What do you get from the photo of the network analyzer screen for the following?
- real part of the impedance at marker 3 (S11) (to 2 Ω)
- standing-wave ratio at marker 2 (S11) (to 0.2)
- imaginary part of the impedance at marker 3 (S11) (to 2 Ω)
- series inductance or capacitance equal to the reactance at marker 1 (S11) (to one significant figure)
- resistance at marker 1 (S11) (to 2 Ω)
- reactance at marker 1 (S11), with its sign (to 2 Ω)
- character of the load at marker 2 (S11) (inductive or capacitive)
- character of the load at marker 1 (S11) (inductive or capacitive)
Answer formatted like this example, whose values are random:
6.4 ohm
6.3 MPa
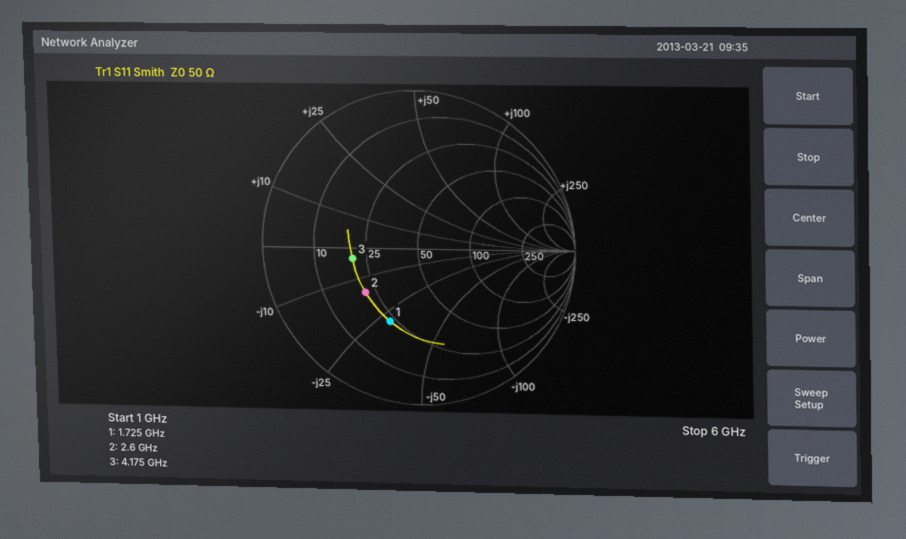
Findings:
20 Ω
2.6
-4 Ω
3 pF
22 Ω
-28 Ω
capacitive
capacitive
